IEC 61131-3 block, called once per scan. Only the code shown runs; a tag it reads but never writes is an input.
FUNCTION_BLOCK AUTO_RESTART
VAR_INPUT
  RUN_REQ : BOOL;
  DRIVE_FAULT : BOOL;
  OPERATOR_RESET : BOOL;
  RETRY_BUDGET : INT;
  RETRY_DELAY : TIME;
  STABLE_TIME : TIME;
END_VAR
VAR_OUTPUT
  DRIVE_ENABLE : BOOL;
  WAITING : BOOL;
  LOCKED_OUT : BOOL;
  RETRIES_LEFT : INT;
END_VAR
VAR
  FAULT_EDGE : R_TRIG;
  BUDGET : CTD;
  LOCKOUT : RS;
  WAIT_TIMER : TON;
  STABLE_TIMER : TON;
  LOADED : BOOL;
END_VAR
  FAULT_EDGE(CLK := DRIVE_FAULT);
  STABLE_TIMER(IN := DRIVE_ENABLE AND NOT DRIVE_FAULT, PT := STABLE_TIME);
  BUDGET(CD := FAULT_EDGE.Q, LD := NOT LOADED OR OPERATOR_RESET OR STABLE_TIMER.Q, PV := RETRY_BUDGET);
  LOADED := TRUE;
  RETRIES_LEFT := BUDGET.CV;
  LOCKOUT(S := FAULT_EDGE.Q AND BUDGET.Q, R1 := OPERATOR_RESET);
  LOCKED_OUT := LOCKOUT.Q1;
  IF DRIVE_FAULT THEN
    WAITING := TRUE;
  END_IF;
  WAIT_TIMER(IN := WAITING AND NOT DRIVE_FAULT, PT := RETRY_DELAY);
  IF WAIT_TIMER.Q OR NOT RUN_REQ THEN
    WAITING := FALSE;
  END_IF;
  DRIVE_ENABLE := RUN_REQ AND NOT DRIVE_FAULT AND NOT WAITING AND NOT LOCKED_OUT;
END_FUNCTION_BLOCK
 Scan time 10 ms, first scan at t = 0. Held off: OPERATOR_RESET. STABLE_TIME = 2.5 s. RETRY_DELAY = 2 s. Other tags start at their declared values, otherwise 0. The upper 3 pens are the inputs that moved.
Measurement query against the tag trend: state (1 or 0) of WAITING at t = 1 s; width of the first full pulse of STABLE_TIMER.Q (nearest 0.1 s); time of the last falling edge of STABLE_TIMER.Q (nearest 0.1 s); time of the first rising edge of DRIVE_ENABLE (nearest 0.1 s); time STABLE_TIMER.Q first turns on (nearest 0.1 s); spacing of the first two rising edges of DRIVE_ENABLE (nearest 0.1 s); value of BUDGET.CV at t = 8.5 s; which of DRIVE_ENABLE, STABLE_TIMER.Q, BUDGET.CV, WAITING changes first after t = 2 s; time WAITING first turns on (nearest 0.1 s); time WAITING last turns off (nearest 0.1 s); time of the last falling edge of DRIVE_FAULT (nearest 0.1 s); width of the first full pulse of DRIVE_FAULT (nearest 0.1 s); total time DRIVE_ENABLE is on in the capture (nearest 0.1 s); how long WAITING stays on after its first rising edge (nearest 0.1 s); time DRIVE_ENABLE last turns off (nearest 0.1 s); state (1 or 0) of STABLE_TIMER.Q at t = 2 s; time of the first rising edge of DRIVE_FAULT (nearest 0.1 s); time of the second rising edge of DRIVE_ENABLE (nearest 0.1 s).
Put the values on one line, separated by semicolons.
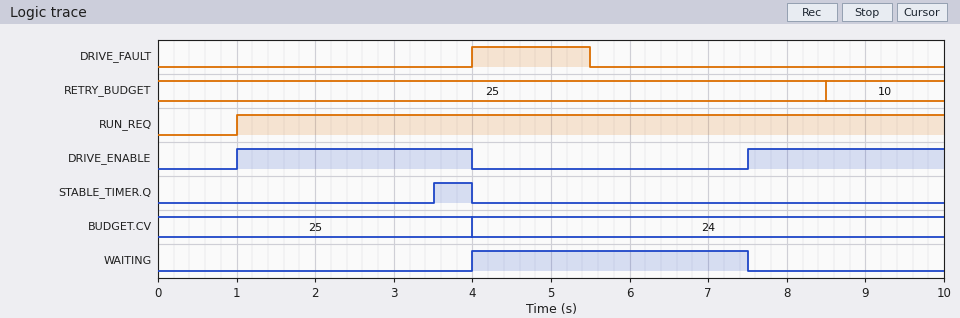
0; 0.5 s; 4.0 s; 1.0 s; 3.5 s; 6.5 s; 24; STABLE_TIMER.Q; 4.0 s; 7.5 s; 5.5 s; 1.5 s; 5.5 s; 3.5 s; 4.0 s; 0; 4.0 s; 7.5 s
